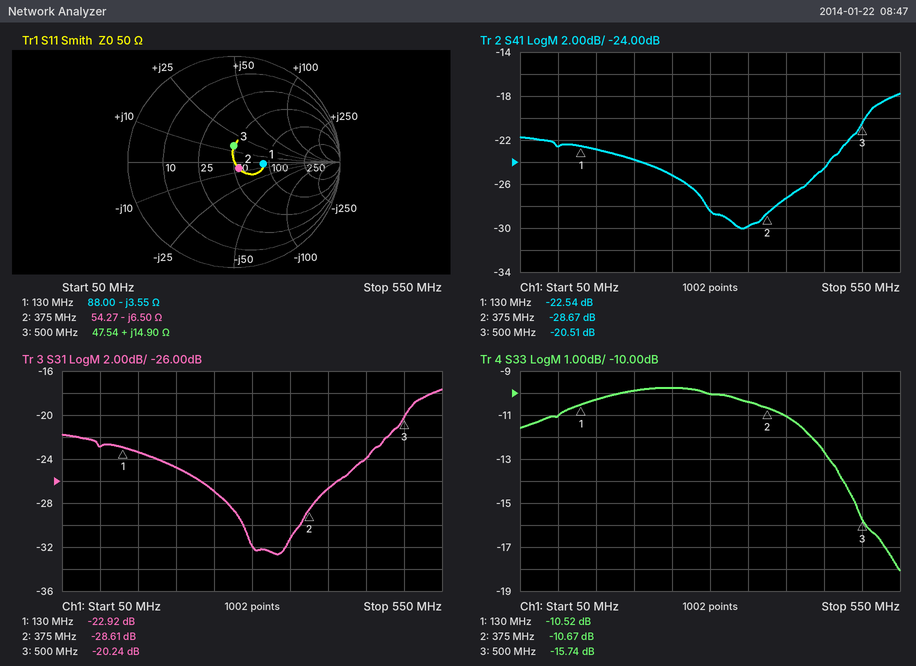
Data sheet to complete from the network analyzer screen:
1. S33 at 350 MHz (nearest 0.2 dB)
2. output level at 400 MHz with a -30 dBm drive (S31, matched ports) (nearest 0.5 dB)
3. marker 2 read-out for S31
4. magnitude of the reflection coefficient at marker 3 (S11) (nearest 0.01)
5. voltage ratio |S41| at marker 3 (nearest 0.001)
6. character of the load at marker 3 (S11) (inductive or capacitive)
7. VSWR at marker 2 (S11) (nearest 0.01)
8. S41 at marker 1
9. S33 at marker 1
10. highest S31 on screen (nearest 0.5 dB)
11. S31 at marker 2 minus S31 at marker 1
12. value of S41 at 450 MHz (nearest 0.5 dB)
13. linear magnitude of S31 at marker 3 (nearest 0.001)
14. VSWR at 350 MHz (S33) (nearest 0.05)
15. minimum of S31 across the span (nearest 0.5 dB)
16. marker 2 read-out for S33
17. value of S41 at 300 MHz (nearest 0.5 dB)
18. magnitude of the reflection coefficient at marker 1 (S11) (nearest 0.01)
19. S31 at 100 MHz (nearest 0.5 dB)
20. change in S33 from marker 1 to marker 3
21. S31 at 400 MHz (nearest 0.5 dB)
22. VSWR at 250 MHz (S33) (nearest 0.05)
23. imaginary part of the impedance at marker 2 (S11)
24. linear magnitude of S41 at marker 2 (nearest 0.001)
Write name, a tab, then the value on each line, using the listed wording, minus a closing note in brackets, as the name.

S33 at 350 MHz	-10.4 dB
output level at 400 MHz with a -30 dBm drive (S31, matched ports)	-56.5 dBm
marker 2 read-out for S31	-28.61 dB
magnitude of the reflection coefficient at marker 3 (S11)	0.15
voltage ratio |S41| at marker 3	0.094
character of the load at marker 3 (S11)	inductive
VSWR at marker 2 (S11)	1.16
S41 at marker 1	-22.54 dB
S33 at marker 1	-10.52 dB
highest S31 on screen	-17.5 dB
S31 at marker 2 minus S31 at marker 1	-5.69 dB
value of S41 at 450 MHz	-24.5 dB
linear magnitude of S31 at marker 3	0.097
VSWR at 350 MHz (S33)	1.85
minimum of S31 across the span	-32.5 dB
marker 2 read-out for S33	-10.67 dB
value of S41 at 300 MHz	-28.5 dB
magnitude of the reflection coefficient at marker 1 (S11)	0.28
S31 at 100 MHz	-23.0 dB
change in S33 from marker 1 to marker 3	-5.22 dB
S31 at 400 MHz	-26.5 dB
VSWR at 250 MHz (S33)	1.95
imaginary part of the impedance at marker 2	-6.50 Ω
linear magnitude of S41 at marker 2	0.037
